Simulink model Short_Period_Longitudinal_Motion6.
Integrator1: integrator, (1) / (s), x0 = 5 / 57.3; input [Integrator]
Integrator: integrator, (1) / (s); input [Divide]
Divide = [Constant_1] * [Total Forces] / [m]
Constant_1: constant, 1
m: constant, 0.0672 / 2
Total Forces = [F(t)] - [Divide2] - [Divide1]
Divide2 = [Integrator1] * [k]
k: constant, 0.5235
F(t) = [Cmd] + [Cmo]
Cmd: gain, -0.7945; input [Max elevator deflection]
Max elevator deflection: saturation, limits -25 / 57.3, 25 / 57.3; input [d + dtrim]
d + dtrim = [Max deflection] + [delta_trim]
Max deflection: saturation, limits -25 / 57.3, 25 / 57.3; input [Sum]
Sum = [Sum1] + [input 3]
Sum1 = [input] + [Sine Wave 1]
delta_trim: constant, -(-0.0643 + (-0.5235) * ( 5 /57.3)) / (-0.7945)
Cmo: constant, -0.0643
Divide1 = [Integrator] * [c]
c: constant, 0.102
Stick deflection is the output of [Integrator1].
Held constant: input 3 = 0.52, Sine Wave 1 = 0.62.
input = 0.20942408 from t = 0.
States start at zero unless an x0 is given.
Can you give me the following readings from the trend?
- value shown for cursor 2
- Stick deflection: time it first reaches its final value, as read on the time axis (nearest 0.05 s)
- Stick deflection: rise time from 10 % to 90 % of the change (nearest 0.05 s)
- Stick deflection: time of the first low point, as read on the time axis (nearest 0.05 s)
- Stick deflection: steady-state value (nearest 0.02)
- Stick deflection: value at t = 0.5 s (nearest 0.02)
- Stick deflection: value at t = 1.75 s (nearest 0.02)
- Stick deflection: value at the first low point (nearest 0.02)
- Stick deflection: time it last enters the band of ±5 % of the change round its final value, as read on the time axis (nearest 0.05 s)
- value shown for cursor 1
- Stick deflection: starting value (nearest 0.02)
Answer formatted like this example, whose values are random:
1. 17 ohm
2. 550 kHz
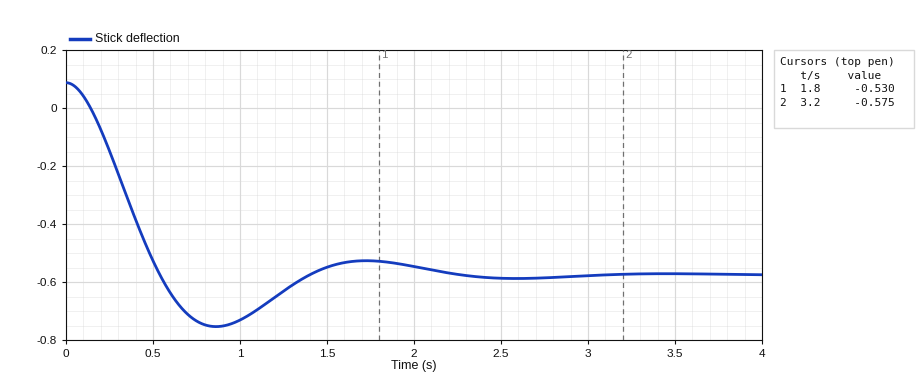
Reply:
1. -0.575
2. 0.55 s
3. 0.35 s
4. 0.85 s
5. -0.58
6. -0.52
7. -0.52
8. -0.76
9. 1.95 s
10. -0.530
11. 0.08
